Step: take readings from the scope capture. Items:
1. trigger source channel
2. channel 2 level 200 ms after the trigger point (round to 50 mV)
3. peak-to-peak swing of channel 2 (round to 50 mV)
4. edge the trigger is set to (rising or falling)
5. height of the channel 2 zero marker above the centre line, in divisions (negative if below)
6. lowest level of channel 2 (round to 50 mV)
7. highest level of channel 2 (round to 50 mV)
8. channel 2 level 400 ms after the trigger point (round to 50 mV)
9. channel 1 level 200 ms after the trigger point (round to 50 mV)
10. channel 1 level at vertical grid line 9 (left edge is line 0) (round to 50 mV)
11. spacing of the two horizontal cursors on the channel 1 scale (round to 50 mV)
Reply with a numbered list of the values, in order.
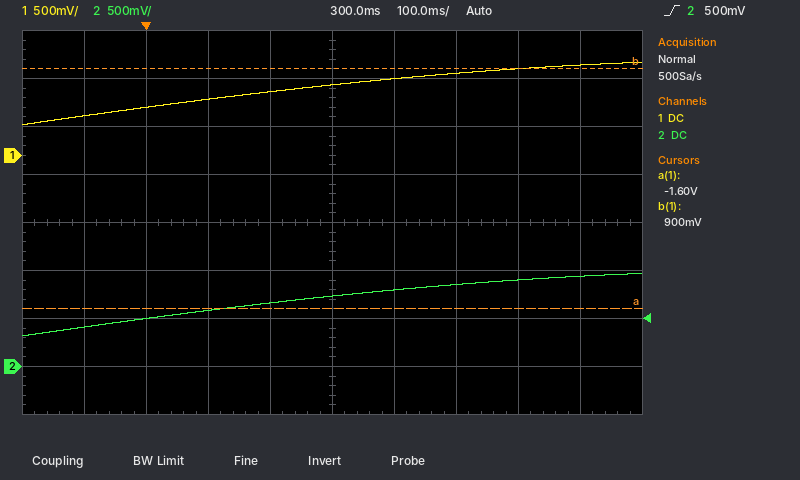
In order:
1. channel 2
2. 650 mV
3. 650 mV
4. rising
5. -3.0 div
6. 300 mV
7. 950 mV
8. 800 mV
9. 650 mV
10. 950 mV
11. 2.50 V
